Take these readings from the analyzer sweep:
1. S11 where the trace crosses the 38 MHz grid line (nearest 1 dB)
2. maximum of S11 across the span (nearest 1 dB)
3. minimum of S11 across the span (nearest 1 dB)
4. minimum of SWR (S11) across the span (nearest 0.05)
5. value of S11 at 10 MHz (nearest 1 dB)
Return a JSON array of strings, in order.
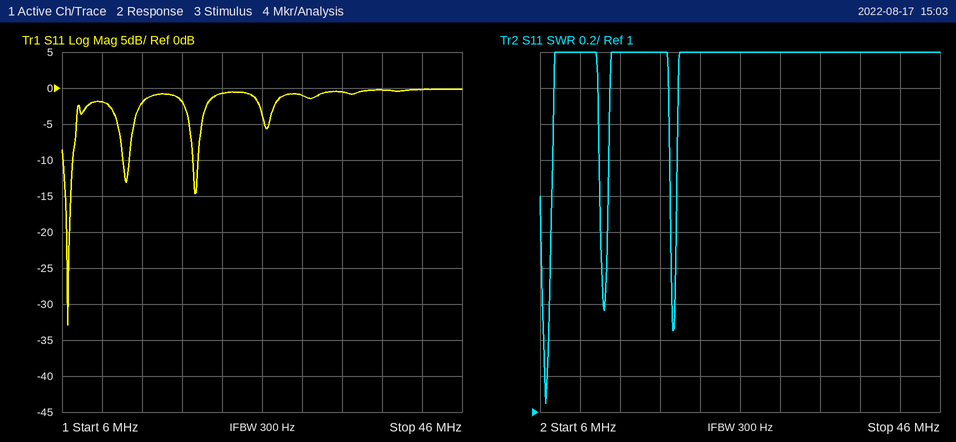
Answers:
["0 dB", "0 dB", "-33 dB", "1.05", "-2 dB"]
